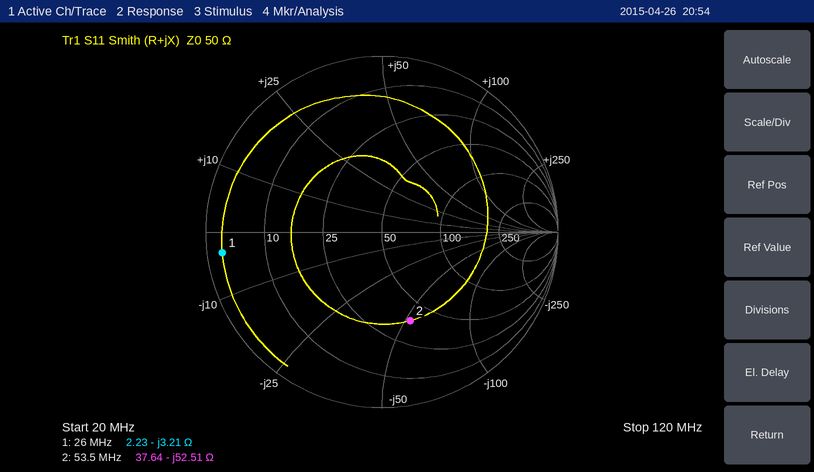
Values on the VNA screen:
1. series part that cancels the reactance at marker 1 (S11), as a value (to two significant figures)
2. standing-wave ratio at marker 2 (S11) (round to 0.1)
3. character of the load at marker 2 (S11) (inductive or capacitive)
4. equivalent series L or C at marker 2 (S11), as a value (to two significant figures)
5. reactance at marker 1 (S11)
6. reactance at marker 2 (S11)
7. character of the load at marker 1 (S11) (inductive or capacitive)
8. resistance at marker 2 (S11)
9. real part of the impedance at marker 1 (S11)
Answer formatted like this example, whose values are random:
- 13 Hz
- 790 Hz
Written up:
- 20 nH
- 3.2
- capacitive
- 57 pF
- -3.21 Ω
- -52.51 Ω
- capacitive
- 37.64 Ω
- 2.23 Ω
